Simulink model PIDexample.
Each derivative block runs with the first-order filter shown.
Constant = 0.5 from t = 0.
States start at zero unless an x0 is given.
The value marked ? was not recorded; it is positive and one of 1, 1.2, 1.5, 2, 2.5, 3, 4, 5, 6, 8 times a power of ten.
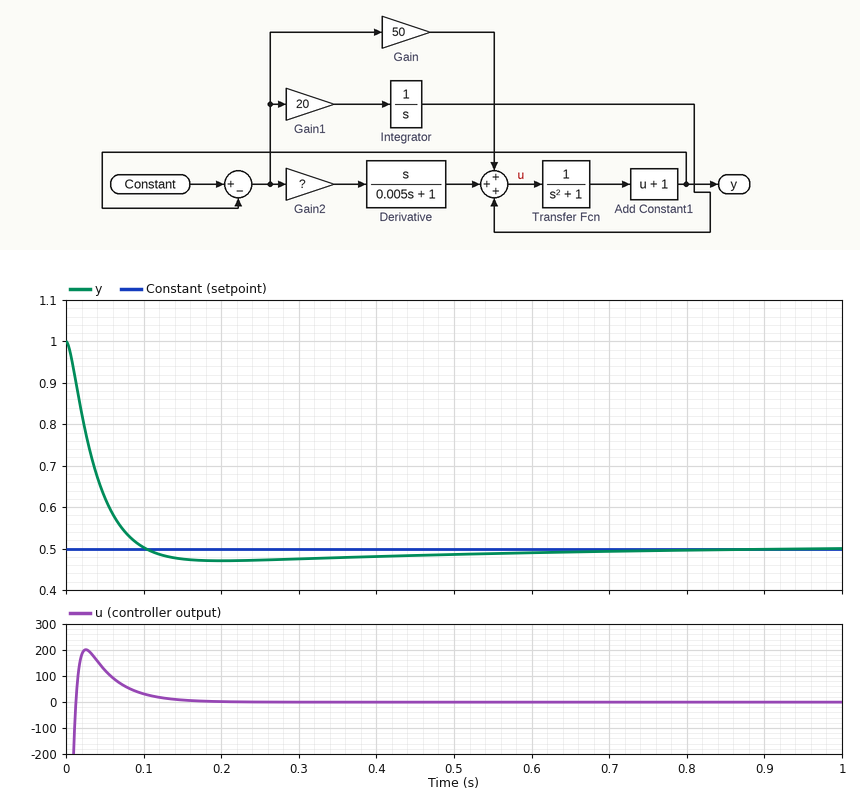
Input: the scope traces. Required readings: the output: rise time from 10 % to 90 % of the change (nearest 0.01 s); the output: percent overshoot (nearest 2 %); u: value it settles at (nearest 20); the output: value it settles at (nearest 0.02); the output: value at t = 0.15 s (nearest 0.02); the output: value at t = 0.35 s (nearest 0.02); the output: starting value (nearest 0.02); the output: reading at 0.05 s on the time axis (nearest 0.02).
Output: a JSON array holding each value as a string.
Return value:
["0.06 s", "6 %", "0", "0.50", "0.48", "0.48", "1.00", "0.62"]
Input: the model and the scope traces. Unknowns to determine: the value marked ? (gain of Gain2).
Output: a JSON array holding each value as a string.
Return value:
["25"]
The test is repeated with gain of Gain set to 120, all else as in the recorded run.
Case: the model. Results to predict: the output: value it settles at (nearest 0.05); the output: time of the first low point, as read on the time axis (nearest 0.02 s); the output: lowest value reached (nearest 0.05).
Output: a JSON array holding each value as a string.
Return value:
["0.50", "0.16 s", "0.45"]
